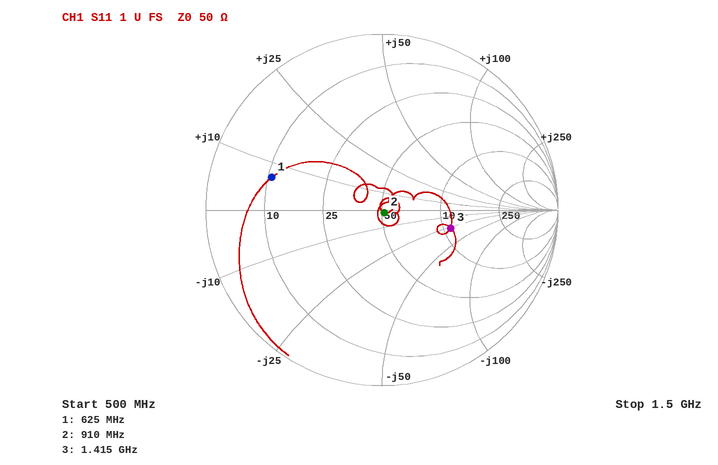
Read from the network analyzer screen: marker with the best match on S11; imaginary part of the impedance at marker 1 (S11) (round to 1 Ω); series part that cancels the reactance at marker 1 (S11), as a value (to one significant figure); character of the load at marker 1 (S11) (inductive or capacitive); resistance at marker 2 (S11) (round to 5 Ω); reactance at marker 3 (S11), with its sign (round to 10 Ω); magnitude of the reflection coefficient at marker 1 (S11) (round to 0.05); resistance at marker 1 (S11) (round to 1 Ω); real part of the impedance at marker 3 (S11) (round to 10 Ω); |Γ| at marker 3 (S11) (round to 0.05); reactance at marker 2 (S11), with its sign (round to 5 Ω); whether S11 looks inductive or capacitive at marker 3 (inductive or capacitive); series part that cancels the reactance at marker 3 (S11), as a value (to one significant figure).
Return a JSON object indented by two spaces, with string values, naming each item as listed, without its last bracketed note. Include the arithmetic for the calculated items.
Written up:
{
  "marker with the best match on S11": "marker 2",
  "imaginary part of the impedance at marker 1 (S11)": "+7 Ω",
  "series part that cancels the reactance at marker 1 (S11), as a value": "C = 1/(2π × 625 MHz × 7 Ω) ≈ 36.4 pF, so 40 pF to one significant figure",
  "character of the load at marker 1 (S11)": "inductive",
  "resistance at marker 2 (S11)": "50 Ω",
  "reactance at marker 3 (S11), with its sign": "-30 Ω",
  "magnitude of the reflection coefficient at marker 1 (S11)": "0.65",
  "resistance at marker 1 (S11)": "11 Ω",
  "real part of the impedance at marker 3 (S11)": "110 Ω",
  "|Γ| at marker 3 (S11)": "0.40",
  "reactance at marker 2 (S11), with its sign": "0 Ω",
  "whether S11 looks inductive or capacitive at marker 3": "capacitive",
  "series part that cancels the reactance at marker 3 (S11), as a value": "L = 30 Ω/(2π × 1.415 GHz) ≈ 3 nH"
}
